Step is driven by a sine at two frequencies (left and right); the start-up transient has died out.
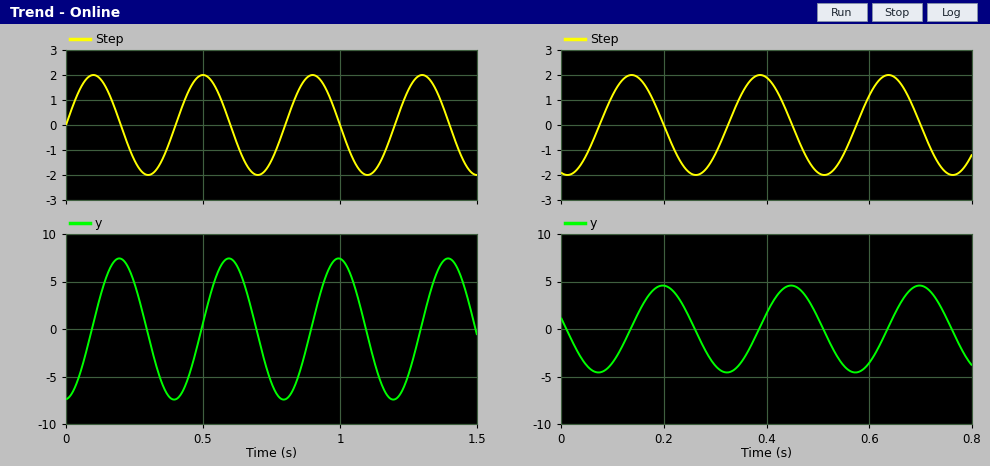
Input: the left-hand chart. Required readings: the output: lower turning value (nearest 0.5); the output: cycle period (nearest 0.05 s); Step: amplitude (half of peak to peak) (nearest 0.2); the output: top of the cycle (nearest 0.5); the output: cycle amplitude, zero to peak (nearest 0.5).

-7.5
0.40 s
2.0
7.5
7.5
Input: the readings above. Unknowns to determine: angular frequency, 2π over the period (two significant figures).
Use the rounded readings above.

16 rad/s
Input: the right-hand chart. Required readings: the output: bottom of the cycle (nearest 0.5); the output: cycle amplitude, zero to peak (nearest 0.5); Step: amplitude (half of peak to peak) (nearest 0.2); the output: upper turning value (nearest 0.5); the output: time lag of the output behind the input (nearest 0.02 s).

-4.5
4.5
2.0
4.5
0.06 s
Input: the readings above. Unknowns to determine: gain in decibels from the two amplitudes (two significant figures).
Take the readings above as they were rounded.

7.0 dB
